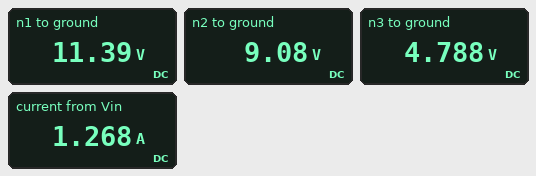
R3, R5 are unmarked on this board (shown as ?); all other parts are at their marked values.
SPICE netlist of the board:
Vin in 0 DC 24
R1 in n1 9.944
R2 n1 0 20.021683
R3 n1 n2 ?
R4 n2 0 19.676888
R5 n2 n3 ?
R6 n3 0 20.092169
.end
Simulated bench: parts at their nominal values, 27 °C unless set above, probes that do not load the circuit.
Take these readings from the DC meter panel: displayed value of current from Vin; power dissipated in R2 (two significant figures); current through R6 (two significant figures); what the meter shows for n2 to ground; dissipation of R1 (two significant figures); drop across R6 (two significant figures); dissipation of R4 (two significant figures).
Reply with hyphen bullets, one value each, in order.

- 1.268 A
- 6.5 W
- 240 mA
- 9.08 V
- 16 W
- 4.8 V
- 4.2 W
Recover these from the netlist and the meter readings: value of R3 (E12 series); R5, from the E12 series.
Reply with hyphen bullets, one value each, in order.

- 3.3 Ω
- 18 Ω
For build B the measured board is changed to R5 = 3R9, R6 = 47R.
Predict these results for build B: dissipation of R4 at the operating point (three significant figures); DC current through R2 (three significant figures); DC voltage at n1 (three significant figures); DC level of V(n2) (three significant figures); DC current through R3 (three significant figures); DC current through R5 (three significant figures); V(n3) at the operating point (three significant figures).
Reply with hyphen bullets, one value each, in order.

- 4.52 W
- 580 mA
- 11.6 V
- 9.43 V
- 664 mA
- 185 mA
- 8.71 V
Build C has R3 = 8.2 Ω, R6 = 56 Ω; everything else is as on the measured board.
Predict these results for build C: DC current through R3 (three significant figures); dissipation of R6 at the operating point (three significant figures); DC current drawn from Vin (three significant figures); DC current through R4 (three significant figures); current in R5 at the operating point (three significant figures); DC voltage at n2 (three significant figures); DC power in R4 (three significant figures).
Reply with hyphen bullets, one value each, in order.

- 528 mA
- 688 mW
- 1.15 A
- 417 mA
- 111 mA
- 8.20 V
- 3.42 W
